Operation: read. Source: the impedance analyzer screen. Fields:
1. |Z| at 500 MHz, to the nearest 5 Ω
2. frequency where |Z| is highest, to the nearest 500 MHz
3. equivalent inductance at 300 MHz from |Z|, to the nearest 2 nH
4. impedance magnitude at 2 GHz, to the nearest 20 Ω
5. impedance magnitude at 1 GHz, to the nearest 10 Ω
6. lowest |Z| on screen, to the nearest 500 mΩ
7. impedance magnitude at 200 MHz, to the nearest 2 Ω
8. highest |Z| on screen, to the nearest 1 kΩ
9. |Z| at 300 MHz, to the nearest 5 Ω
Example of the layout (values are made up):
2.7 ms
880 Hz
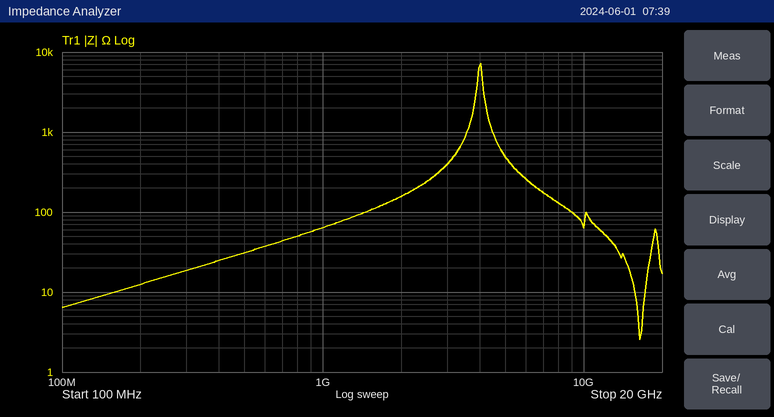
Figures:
30 Ω
4.0 GHz
10 nH
160 Ω
60 Ω
2.5 Ω
12 Ω
7 kΩ
20 Ω
